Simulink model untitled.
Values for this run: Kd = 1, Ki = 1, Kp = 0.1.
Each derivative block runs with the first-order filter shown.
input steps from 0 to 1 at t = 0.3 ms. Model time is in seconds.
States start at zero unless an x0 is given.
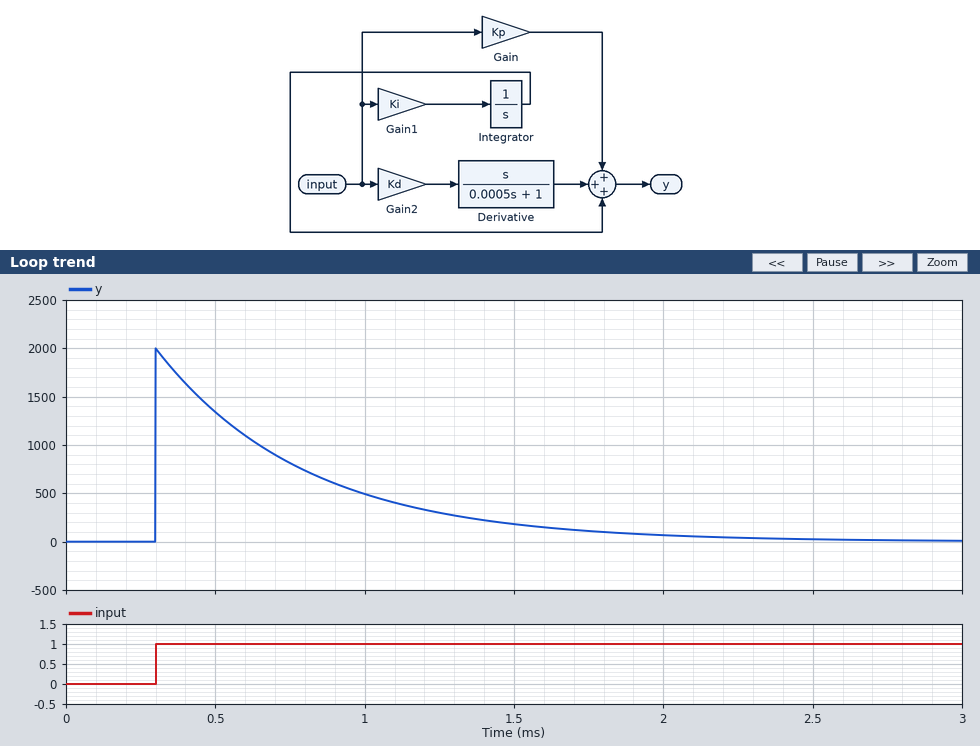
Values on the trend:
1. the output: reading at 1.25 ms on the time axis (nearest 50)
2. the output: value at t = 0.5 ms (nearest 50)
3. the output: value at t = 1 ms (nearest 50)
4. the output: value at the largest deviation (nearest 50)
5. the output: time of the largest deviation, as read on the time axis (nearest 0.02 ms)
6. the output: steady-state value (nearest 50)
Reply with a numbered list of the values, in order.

1. 300
2. 1350
3. 500
4. 2000
5. 0.30 ms
6. 0
